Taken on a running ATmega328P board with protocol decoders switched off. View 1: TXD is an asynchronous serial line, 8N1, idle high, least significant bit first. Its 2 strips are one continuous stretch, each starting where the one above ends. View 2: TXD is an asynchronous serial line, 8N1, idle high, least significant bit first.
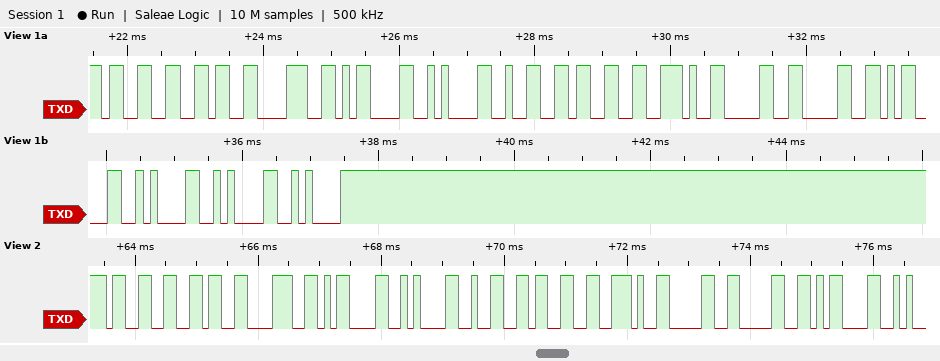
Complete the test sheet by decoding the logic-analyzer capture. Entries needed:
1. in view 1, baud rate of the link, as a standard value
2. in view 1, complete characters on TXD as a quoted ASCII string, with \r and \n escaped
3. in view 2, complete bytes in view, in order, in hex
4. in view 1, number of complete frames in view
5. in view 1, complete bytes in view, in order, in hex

9600 baud
"368\r\n23.00\r\n\n\n"
33 36 38 0D 0A 32 33 2E 30 30 0D
14
33 36 38 0D 0A 32 33 2E 30 30 0D 0A 0A 0A
